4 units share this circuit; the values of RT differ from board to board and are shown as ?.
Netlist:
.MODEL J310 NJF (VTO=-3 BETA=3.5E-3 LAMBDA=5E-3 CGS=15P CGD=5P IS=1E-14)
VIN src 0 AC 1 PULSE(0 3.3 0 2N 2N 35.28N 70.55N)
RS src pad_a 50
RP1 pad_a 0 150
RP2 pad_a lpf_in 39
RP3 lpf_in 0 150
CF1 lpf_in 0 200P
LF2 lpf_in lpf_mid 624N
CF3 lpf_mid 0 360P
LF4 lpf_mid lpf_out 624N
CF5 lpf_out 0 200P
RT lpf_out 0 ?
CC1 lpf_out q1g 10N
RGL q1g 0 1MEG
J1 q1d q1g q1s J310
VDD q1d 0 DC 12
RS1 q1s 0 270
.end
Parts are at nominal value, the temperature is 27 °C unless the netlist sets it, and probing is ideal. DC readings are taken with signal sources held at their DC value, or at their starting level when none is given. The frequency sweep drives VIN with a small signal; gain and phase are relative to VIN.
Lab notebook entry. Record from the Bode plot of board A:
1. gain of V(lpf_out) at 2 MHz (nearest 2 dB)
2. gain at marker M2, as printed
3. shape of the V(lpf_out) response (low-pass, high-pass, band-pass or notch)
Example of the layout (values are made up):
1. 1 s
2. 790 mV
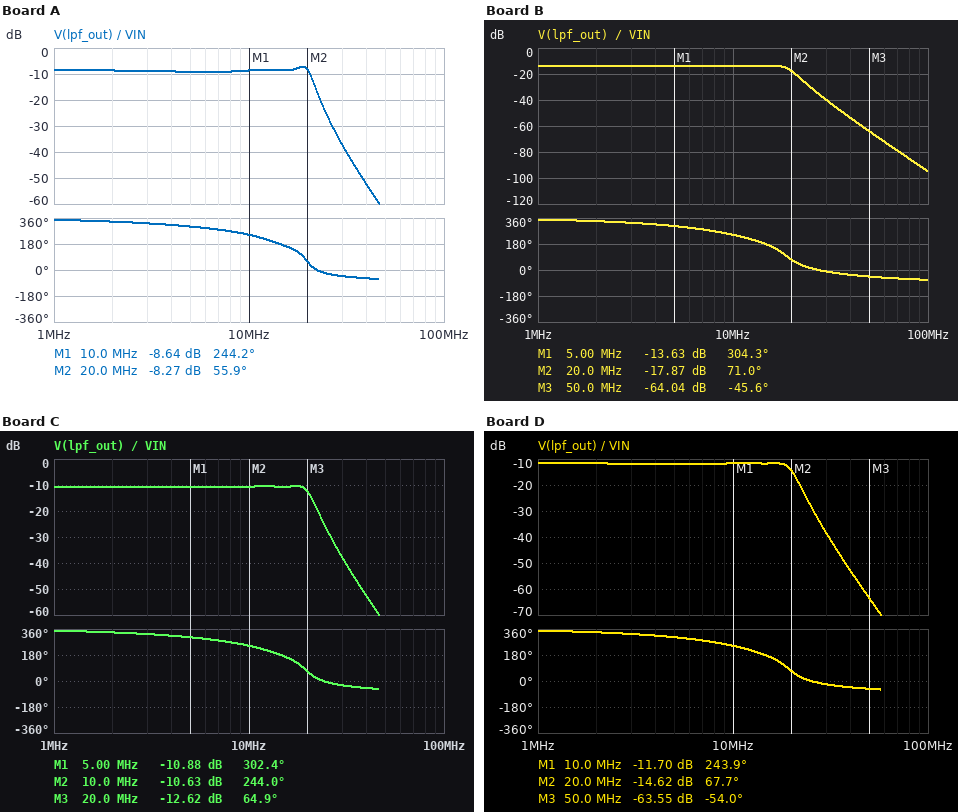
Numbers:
1. -8 dB
2. -8.27 dB
3. low-pass
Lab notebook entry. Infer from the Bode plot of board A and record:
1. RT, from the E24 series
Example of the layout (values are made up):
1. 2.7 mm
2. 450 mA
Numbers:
1. 160 Ω
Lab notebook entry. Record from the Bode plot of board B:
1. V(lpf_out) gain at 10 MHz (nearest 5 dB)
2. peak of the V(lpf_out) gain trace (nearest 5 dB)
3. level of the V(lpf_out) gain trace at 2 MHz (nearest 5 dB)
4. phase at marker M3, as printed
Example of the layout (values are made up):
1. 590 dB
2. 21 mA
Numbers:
1. -15 dB
2. -15 dB
3. -15 dB
4. -45.6 deg
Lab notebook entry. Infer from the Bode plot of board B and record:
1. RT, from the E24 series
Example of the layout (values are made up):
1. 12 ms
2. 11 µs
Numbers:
1. 36 Ω
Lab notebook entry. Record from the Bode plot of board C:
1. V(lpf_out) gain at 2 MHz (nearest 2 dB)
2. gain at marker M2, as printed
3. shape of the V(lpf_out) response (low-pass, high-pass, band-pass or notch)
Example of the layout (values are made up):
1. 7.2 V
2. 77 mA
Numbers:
1. -10 dB
2. -10.63 dB
3. low-pass
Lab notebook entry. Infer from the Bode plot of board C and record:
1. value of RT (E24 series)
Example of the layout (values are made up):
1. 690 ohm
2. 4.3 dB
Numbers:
1. 75 Ω
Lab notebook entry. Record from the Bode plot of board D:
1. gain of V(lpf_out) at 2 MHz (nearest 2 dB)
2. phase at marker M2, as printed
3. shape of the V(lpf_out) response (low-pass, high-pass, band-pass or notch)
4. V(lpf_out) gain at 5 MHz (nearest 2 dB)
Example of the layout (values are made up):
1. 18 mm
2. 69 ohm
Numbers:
1. -12 dB
2. 67.7 deg
3. low-pass
4. -12 dB
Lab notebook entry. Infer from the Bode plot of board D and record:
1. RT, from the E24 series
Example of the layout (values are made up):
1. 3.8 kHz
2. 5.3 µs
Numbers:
1. 56 Ω
